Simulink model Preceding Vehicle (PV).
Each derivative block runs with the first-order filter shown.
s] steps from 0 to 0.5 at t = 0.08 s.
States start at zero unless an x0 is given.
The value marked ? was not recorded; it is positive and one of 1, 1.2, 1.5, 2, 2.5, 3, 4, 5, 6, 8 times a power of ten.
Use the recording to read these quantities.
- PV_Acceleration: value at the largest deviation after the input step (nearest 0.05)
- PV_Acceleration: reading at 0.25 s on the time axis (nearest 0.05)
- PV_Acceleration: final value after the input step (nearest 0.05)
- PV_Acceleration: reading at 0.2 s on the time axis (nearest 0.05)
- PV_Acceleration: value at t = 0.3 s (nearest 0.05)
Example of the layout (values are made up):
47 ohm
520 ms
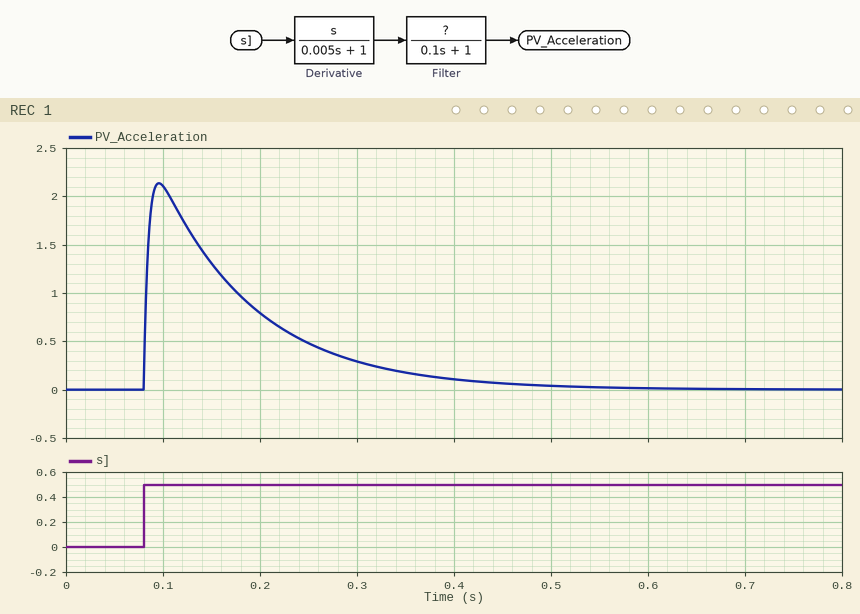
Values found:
2.15
0.50
0.00
0.80
0.30
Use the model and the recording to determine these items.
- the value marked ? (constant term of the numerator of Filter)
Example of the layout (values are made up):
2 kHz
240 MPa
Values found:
0.5
